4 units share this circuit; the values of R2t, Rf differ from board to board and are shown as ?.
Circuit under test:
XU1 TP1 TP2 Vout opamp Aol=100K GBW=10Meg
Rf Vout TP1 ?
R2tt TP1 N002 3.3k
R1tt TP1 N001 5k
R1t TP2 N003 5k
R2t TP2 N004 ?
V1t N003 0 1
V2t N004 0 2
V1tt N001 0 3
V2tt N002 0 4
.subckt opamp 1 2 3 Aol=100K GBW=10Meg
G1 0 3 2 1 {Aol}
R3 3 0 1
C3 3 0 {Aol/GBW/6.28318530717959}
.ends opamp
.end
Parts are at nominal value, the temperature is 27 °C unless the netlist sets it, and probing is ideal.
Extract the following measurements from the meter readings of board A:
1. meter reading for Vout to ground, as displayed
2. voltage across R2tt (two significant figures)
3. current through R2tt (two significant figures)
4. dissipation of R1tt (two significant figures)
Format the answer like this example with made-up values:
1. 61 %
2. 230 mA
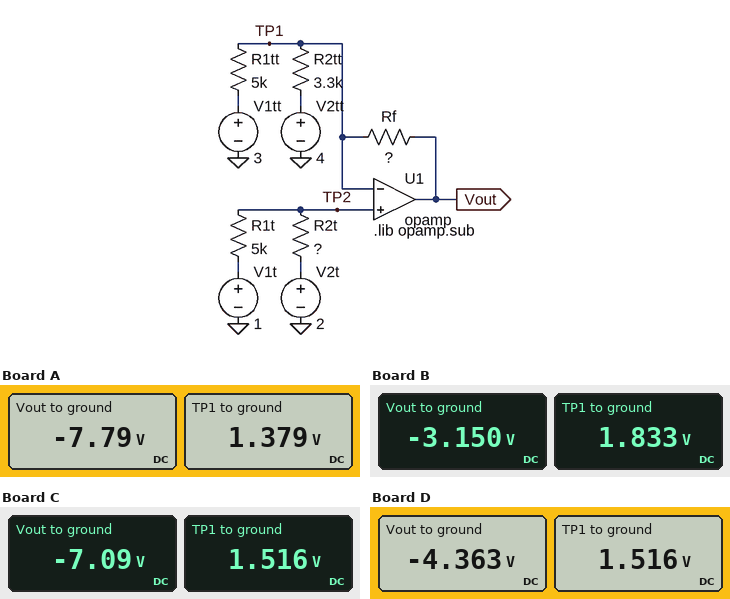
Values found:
1. -7.79 V
2. 2.6 V
3. 790 µA
4. 530 µW
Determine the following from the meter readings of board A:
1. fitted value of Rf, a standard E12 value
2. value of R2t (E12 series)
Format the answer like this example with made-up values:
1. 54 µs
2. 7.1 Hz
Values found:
1. 8.2 kΩ
2. 8.2 kΩ
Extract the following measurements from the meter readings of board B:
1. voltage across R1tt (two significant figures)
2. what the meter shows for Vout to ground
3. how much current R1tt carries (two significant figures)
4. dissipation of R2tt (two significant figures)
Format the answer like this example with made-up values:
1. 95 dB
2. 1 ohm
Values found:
1. 1.2 V
2. -3.150 V
3. 230 µA
4. 1.4 mW
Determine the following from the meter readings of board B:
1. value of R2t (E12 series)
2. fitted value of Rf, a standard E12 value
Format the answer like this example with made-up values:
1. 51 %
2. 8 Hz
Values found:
1. 1 kΩ
2. 5.6 kΩ
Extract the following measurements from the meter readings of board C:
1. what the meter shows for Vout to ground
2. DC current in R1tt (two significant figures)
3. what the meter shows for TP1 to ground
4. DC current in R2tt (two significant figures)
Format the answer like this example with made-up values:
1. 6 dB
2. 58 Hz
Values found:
1. -7.09 V
2. 300 µA
3. 1.516 V
4. 750 µA
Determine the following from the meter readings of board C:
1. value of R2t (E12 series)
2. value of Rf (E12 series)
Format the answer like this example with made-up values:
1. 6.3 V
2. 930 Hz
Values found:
1. 4.7 kΩ
2. 8.2 kΩ
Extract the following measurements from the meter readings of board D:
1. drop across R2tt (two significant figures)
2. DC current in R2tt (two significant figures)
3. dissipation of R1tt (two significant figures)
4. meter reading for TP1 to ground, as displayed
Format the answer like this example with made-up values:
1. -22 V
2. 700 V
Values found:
1. 2.5 V
2. 750 µA
3. 440 µW
4. 1.516 V
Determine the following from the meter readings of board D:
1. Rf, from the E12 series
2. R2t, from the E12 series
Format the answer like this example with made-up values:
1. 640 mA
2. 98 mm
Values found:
1. 5.6 kΩ
2. 4.7 kΩ
